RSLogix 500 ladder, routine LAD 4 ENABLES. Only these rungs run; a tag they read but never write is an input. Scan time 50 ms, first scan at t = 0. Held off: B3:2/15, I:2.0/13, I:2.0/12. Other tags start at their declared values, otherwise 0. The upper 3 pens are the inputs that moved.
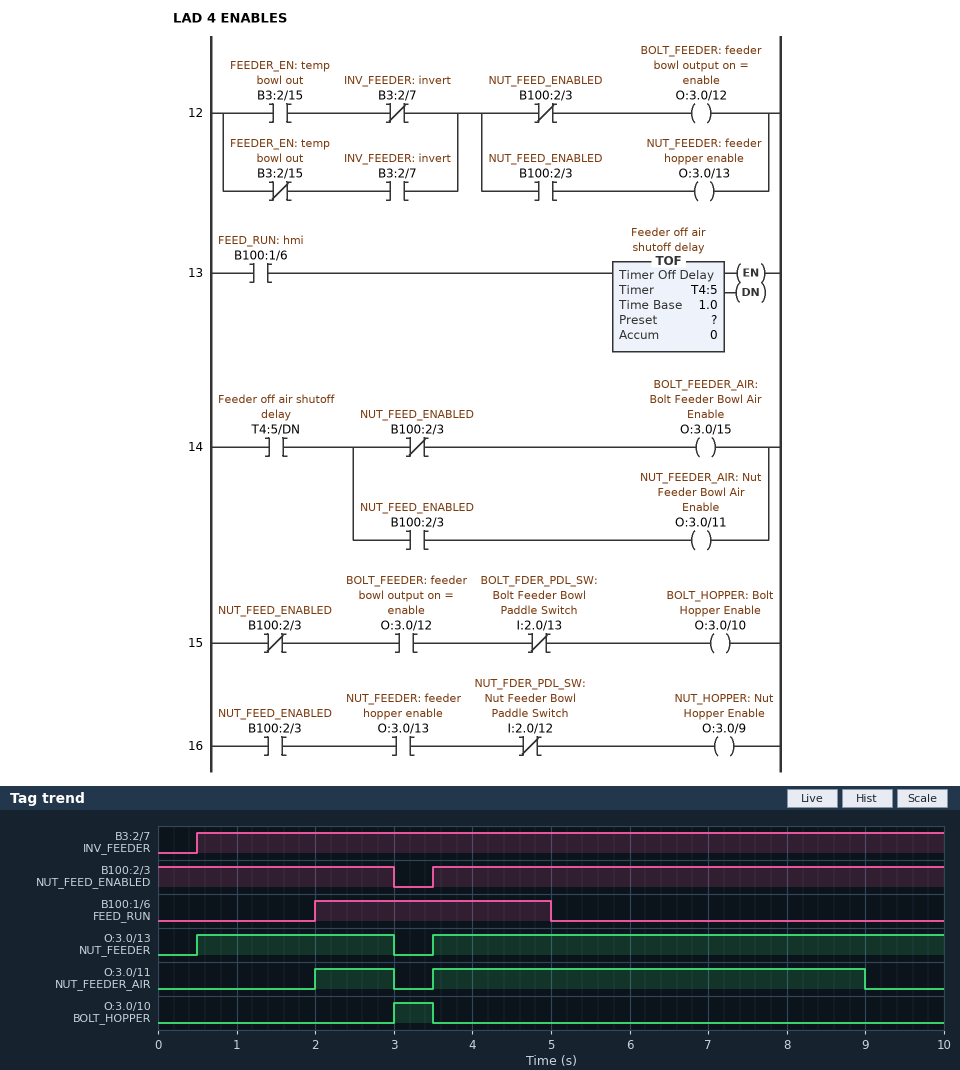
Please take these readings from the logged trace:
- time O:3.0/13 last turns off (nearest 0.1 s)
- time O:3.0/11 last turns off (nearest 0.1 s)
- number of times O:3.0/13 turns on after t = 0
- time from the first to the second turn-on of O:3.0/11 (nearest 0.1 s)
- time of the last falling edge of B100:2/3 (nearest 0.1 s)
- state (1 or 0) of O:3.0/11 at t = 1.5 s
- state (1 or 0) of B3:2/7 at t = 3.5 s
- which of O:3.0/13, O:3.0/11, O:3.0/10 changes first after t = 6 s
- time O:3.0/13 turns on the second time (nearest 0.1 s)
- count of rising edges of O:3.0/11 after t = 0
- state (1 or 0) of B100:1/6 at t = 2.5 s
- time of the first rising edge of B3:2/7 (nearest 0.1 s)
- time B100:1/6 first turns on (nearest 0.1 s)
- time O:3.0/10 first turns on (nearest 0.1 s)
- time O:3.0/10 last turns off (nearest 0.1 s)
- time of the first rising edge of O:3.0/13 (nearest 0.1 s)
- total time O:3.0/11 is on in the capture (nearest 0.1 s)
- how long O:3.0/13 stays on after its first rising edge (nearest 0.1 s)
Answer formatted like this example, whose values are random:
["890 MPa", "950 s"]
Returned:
["3.0 s", "9.0 s", "2", "1.5 s", "3.0 s", "0", "1", "O:3.0/11", "3.5 s", "2", "1", "0.5 s", "2.0 s", "3.0 s", "3.5 s", "0.5 s", "6.5 s", "2.5 s"]
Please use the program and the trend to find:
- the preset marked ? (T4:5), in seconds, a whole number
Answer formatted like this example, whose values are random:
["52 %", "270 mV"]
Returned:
["4 s"]
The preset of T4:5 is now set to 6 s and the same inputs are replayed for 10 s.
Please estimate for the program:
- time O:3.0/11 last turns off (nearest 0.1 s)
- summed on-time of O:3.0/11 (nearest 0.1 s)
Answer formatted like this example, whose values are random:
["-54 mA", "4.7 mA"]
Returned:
["3.0 s", "7.5 s"]
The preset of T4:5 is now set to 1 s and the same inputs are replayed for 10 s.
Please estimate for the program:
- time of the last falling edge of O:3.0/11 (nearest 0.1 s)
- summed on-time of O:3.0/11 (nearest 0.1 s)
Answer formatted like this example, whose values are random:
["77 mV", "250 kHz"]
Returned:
["6.0 s", "3.5 s"]
